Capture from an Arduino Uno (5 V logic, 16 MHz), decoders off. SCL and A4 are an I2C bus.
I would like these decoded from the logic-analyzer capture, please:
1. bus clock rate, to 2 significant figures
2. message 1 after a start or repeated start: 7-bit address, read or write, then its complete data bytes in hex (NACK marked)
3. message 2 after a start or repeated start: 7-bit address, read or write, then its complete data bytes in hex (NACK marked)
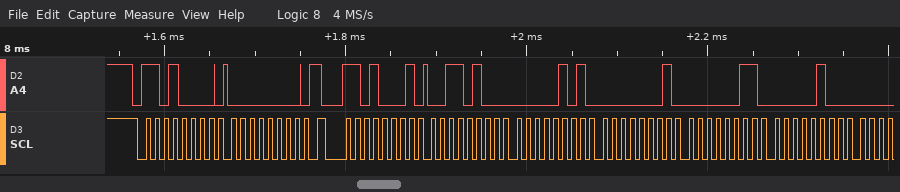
100 kHz
0x68 write: 00
0x68 read: 34 05 01 03 04
